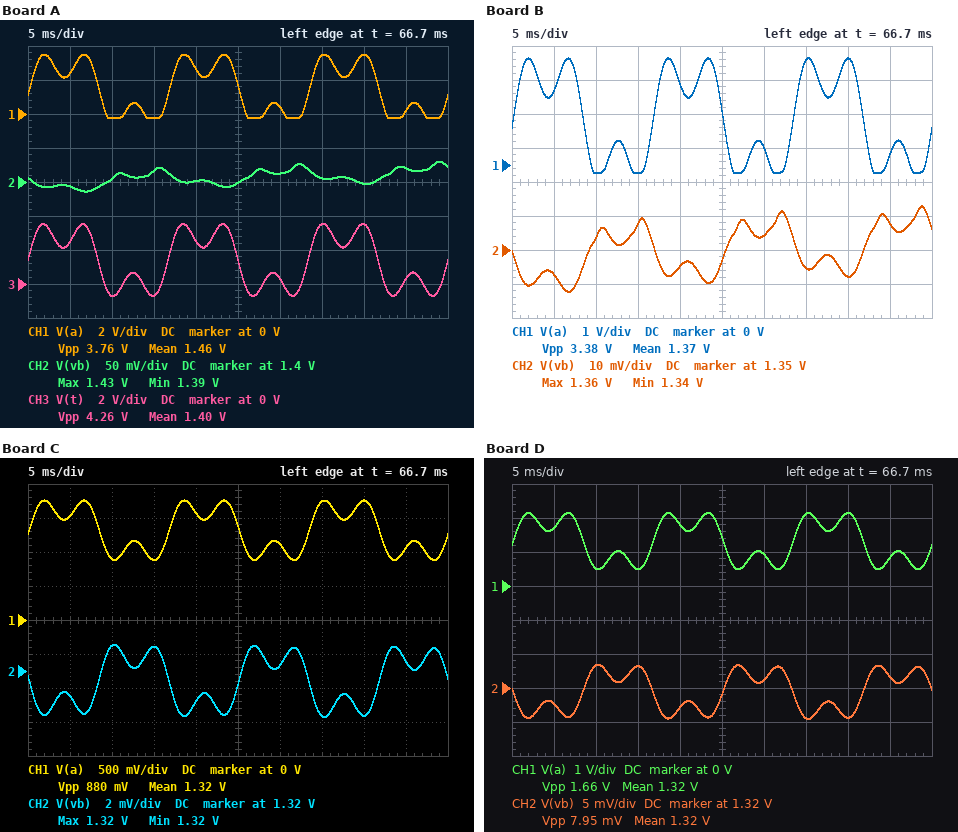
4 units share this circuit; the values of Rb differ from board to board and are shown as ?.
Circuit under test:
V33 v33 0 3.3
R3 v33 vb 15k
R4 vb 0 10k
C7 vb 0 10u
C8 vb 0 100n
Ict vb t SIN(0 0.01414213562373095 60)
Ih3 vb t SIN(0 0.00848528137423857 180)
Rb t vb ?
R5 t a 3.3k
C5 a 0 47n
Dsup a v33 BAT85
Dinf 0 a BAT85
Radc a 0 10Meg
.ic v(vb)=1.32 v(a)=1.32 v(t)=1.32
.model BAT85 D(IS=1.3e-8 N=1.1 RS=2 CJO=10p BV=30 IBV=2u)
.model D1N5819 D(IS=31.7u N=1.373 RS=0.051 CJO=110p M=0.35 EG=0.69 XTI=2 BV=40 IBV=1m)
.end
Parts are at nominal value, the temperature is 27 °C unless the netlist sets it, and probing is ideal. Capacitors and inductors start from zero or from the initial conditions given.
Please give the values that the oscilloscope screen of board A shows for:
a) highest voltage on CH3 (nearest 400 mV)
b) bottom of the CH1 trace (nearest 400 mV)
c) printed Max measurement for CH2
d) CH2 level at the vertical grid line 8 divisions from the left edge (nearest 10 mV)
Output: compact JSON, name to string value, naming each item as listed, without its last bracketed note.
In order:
{"highest voltage on CH3": "3.6 V", "bottom of the CH1 trace": "-400 mV", "printed Max measurement for CH2": "1.43 V", "CH2 level at the vertical grid line 8 divisions from the left edge": "1.40 V"}
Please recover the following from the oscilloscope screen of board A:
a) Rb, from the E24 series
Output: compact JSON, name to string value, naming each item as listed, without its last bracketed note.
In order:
{"Rb, from the E24 series": "130 Ω"}
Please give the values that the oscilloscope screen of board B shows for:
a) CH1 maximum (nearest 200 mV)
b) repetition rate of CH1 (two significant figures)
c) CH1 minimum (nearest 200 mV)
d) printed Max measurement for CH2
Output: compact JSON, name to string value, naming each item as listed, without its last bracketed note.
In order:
{"CH1 maximum": "3.2 V", "repetition rate of CH1": "60 Hz", "CH1 minimum": "-200 mV", "printed Max measurement for CH2": "1.36 V"}
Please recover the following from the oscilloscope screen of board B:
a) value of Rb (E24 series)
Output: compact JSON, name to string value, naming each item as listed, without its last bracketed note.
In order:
{"value of Rb": "110 Ω"}
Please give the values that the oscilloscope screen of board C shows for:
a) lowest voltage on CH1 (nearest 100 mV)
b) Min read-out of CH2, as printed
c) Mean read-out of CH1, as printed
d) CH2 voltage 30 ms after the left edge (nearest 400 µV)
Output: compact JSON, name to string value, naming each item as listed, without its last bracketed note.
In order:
{"lowest voltage on CH1": "900 mV", "Min read-out of CH2, as printed": "1.32 V", "Mean read-out of CH1, as printed": "1.32 V", "CH2 voltage 30 ms after the left edge": "1.3204 V"}
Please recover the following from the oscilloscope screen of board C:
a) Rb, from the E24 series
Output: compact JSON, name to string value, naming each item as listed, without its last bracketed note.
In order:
{"Rb, from the E24 series": "27 Ω"}
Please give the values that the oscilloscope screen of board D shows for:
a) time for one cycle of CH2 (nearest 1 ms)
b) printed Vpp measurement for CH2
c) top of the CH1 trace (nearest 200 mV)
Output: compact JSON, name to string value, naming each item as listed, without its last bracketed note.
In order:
{"time for one cycle of CH2": "17 ms", "printed Vpp measurement for CH2": "7.95 mV", "top of the CH1 trace": "2.2 V"}
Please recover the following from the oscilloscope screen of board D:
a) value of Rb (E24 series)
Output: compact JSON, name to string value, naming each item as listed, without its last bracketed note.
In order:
{"value of Rb": "51 Ω"}
